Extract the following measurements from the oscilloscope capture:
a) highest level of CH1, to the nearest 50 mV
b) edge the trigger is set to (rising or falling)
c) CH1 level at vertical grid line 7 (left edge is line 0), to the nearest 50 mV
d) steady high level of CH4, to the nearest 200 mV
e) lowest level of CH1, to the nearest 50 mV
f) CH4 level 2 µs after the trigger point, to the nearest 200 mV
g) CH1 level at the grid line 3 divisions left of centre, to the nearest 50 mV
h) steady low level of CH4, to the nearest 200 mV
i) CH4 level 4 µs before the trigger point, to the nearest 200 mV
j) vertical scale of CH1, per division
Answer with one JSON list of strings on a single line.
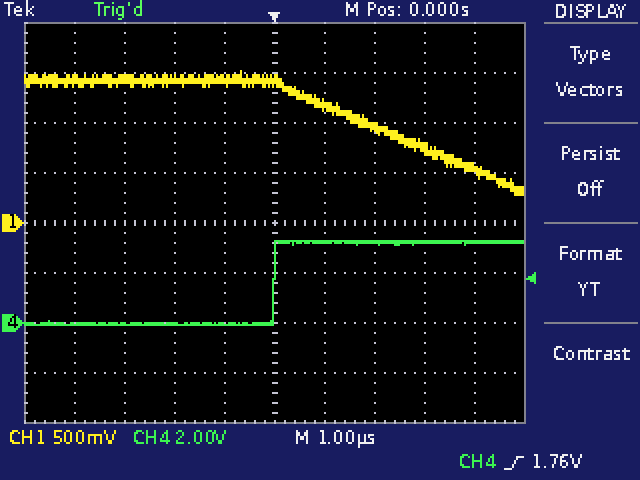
["1.50 V", "rising", "950 mV", "3.2 V", "300 mV", "3.2 V", "1.45 V", "0.0 V", "0.0 V", "500 mV"]
